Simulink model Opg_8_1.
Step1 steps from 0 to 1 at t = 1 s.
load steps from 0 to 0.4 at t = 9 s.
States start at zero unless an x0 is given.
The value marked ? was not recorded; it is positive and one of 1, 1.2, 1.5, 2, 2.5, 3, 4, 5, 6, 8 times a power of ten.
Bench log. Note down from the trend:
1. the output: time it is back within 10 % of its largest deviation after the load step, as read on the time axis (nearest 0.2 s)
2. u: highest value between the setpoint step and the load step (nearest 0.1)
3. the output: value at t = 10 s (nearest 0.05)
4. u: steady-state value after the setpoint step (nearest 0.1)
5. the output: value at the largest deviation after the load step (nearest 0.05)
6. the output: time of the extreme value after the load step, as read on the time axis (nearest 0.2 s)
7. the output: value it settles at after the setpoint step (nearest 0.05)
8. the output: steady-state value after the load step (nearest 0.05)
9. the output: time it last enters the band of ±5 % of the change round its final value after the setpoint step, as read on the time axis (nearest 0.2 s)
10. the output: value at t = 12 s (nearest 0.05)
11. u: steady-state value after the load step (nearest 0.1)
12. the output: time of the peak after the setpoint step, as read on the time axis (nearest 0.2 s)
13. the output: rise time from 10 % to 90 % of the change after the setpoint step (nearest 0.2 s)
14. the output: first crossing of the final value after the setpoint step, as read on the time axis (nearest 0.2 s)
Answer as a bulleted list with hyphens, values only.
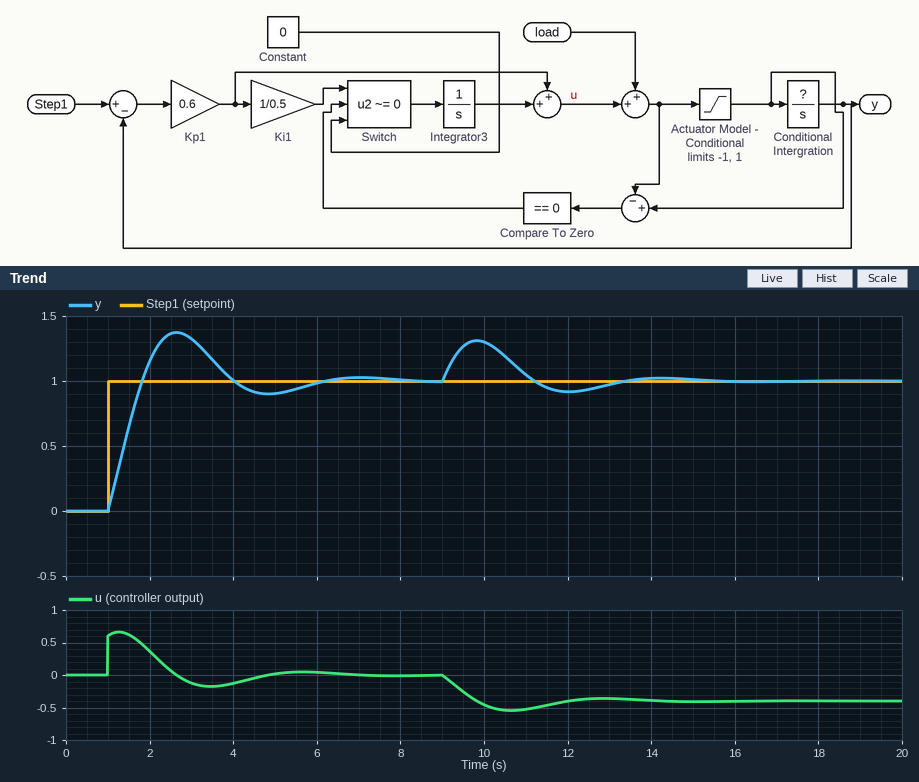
- 13.0 s
- 0.7
- 1.30
- 0.0
- 1.30
- 9.8 s
- 1.00
- 1.00
- 5.6 s
- 0.90
- -0.4
- 2.6 s
- 0.6 s
- 1.8 s
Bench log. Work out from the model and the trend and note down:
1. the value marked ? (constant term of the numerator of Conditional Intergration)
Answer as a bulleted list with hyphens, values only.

- 2
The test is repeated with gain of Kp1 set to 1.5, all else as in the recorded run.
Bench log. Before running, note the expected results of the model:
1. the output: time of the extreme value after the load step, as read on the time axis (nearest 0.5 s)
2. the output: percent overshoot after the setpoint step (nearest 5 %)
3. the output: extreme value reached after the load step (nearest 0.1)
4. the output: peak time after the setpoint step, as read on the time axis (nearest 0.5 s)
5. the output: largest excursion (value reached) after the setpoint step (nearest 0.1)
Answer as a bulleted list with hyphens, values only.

- 9.5 s
- 15 %
- 1.2
- 2.0 s
- 1.2
